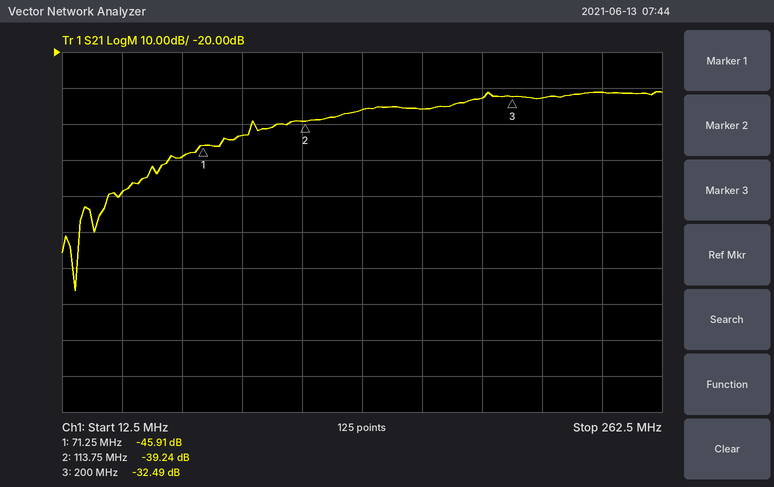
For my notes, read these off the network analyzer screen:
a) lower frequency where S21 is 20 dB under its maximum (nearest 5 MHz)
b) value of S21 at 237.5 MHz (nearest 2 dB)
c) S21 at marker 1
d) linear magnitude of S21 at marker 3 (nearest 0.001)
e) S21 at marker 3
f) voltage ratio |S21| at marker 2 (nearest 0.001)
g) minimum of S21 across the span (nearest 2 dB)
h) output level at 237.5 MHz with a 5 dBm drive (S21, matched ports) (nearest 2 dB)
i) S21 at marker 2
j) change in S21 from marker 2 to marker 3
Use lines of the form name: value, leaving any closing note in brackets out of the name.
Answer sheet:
lower frequency where S21 is 20 dB under its maximum: 55 MHz
value of S21 at 237.5 MHz: -32 dB
S21 at marker 1: -45.91 dB
linear magnitude of S21 at marker 3: 0.024
S21 at marker 3: -32.49 dB
voltage ratio |S21| at marker 2: 0.011
minimum of S21 across the span: -86 dB
output level at 237.5 MHz with a 5 dBm drive (S21, matched ports): -26 dBm
S21 at marker 2: -39.24 dB
change in S21 from marker 2 to marker 3: 6.75 dB
